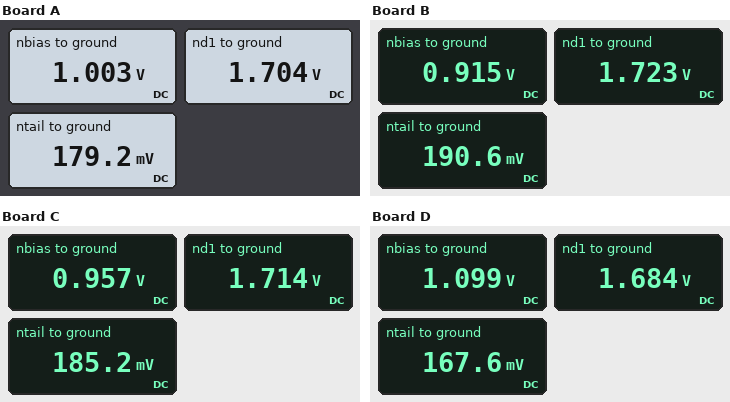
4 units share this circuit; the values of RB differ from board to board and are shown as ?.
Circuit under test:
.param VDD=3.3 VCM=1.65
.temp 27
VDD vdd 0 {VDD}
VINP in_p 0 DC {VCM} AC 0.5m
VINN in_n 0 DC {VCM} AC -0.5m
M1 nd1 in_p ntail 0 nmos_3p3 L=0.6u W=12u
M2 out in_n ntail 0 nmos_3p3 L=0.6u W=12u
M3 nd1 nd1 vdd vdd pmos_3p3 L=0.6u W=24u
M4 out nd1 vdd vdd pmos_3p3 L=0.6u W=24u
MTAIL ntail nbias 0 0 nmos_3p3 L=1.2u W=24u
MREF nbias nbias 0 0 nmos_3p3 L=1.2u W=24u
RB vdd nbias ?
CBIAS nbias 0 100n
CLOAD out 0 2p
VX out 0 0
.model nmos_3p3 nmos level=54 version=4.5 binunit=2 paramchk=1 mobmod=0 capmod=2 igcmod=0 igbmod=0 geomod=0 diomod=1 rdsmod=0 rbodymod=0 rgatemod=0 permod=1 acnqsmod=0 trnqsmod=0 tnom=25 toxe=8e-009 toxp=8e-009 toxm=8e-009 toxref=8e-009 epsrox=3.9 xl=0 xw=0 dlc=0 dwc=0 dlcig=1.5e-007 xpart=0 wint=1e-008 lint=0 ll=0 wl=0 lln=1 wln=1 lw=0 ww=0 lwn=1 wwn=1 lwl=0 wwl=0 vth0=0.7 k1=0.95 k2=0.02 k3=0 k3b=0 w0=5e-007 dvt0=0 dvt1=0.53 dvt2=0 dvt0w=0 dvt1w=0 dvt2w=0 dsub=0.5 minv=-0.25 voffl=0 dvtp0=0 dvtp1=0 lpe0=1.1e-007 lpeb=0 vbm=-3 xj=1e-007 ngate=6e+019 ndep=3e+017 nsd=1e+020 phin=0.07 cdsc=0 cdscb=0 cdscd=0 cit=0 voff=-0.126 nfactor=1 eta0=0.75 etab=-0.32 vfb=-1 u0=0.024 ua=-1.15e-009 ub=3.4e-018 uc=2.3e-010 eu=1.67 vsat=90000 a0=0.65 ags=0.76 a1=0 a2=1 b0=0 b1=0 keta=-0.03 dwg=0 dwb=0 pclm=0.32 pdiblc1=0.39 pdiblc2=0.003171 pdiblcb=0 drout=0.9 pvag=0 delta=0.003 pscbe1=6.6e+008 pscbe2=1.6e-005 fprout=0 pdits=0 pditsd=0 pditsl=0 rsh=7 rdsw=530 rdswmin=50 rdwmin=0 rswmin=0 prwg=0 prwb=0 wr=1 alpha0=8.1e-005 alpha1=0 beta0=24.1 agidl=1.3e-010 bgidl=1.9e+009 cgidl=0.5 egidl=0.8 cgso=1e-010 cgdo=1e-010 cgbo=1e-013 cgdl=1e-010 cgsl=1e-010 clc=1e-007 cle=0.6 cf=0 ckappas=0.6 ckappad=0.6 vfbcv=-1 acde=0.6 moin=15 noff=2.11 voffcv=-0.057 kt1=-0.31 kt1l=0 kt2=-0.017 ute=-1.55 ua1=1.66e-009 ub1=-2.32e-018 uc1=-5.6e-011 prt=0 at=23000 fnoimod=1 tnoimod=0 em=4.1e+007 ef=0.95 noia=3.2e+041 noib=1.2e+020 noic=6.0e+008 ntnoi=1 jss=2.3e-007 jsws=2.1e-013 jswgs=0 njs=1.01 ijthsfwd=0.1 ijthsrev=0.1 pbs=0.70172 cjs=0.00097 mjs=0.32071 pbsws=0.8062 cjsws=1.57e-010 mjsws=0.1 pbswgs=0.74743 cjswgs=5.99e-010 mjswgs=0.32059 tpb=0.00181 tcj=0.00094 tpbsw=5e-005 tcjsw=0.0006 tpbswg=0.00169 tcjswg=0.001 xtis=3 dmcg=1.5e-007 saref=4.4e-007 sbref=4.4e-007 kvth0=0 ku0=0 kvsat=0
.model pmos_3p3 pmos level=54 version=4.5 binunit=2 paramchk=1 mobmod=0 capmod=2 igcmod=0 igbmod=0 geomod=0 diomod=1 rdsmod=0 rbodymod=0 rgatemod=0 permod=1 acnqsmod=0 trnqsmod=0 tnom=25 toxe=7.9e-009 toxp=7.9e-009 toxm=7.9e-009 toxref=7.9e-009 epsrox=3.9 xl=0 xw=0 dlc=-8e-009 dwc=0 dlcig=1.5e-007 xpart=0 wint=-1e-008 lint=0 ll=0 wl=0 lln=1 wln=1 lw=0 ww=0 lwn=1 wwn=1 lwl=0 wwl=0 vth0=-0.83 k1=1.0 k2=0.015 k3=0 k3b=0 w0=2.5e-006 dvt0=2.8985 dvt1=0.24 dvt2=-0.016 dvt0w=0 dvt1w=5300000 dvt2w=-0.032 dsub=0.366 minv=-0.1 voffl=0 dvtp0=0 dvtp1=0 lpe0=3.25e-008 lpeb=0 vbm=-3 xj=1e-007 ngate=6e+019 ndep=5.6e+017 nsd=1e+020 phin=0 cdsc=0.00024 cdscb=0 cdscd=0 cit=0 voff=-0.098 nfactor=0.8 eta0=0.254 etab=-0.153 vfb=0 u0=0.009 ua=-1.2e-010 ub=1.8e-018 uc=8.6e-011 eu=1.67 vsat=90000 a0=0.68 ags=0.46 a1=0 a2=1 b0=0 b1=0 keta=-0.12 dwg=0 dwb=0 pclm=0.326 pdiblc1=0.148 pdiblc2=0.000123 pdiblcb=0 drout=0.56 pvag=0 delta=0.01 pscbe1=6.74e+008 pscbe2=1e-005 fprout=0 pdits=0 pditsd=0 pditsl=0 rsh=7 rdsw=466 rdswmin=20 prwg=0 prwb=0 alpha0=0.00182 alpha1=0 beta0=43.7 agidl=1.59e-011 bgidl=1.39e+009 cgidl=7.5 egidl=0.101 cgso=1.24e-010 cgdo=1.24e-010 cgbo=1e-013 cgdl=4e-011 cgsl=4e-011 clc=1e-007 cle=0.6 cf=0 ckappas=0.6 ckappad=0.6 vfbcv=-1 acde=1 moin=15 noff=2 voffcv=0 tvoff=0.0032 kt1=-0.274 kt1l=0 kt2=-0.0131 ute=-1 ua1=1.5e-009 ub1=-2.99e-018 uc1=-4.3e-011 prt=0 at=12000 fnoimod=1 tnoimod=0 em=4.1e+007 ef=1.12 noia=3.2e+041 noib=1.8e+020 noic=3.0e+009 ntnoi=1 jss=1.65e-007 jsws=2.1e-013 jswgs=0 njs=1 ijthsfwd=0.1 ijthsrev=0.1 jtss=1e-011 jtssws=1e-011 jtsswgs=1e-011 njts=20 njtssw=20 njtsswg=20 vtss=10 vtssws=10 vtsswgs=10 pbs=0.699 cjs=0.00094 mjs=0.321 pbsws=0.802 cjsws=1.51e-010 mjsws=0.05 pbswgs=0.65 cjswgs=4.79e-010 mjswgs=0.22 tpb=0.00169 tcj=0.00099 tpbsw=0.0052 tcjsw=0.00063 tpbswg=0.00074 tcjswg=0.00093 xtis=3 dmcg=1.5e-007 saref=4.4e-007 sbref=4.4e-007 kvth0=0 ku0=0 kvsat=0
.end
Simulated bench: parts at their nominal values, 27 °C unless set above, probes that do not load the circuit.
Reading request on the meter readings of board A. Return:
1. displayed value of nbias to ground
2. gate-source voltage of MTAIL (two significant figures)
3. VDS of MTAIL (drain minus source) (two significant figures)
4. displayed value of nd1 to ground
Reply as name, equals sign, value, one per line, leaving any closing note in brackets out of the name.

displayed value of nbias to ground = 1.003 V
gate-source voltage of MTAIL = 1.0 V
VDS of MTAIL (drain minus source) = 180 mV
displayed value of nd1 to ground = 1.704 V
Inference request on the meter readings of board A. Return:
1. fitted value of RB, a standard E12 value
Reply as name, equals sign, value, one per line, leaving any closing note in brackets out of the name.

fitted value of RB, a standard E12 value = 33 kΩ
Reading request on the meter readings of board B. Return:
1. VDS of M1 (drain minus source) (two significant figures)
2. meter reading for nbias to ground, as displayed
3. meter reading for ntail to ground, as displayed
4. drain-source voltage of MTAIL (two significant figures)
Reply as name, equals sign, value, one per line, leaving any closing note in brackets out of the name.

VDS of M1 (drain minus source) = 1.5 V
meter reading for nbias to ground, as displayed = 0.915 V
meter reading for ntail to ground, as displayed = 190.6 mV
drain-source voltage of MTAIL = 190 mV
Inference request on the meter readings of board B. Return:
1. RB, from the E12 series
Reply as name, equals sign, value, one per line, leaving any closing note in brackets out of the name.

RB, from the E12 series = 68 kΩ
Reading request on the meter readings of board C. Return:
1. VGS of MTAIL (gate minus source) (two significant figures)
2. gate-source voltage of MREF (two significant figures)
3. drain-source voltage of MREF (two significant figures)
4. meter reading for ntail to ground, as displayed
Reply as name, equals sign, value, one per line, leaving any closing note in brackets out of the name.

VGS of MTAIL (gate minus source) = 960 mV
gate-source voltage of MREF = 960 mV
drain-source voltage of MREF = 960 mV
meter reading for ntail to ground, as displayed = 185.2 mV
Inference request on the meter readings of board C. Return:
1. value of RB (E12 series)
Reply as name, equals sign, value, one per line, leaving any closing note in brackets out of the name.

value of RB = 47 kΩ
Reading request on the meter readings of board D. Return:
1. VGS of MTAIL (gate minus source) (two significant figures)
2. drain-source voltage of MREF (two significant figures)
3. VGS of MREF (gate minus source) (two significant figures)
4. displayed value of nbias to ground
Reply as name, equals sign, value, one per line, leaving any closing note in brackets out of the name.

VGS of MTAIL (gate minus source) = 1.1 V
drain-source voltage of MREF = 1.1 V
VGS of MREF (gate minus source) = 1.1 V
displayed value of nbias to ground = 1.099 V
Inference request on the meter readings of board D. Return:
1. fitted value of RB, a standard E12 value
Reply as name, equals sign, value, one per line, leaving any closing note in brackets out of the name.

fitted value of RB, a standard E12 value = 18 kΩ
